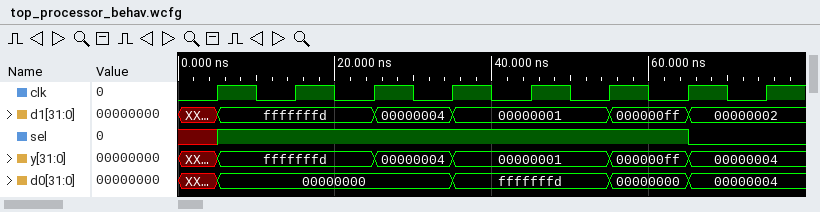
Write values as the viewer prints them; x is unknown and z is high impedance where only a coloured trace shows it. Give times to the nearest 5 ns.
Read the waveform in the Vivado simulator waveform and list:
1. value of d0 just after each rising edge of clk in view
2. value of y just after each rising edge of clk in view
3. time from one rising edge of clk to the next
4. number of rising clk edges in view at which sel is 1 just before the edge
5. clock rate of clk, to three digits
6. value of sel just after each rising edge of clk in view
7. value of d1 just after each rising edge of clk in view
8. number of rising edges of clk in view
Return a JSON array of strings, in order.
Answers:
["00000000, 00000000, 00000000, fffffffd, fffffffd, 00000000, 00000004, 00000004", "fffffffd, fffffffd, 00000004, 00000001, 00000001, 000000ff, 00000004, 00000004", "10 ns", "6", "100 MHz", "1 1 1 1 1 1 0 0", "fffffffd, fffffffd, 00000004, 00000001, 00000001, 000000ff, 00000002, 00000002", "8"]
